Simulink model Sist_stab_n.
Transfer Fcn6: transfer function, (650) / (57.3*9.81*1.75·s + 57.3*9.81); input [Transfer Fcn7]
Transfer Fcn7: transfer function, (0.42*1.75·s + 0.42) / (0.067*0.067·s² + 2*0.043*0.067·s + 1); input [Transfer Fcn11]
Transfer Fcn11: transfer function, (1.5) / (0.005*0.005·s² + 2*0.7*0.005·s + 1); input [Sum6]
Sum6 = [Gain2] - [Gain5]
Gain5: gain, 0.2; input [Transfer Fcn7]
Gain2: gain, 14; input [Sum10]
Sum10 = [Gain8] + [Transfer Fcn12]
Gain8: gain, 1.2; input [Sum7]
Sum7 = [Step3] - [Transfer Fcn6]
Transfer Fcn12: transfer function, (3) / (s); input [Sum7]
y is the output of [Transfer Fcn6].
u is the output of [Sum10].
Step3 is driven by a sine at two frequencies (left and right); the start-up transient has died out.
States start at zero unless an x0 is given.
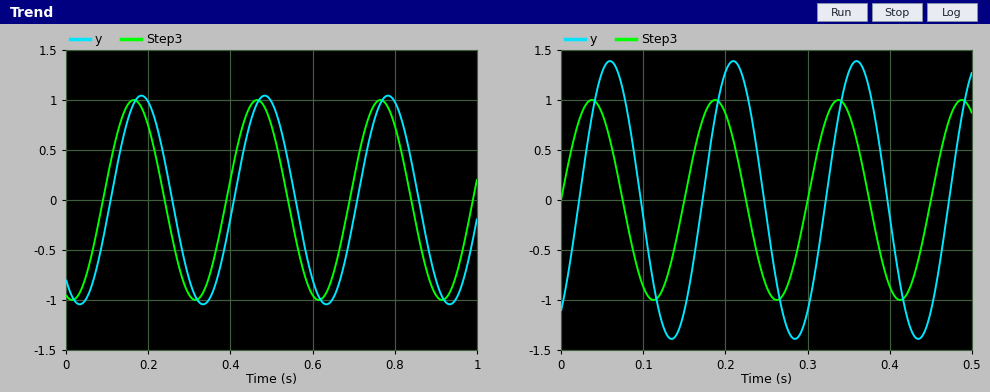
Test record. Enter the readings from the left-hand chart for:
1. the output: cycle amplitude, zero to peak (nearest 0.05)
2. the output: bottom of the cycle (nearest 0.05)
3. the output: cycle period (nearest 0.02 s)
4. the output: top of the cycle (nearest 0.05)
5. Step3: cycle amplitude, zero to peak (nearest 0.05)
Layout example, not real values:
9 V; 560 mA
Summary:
1.05; -1.05; 0.30 s; 1.05; 1.00
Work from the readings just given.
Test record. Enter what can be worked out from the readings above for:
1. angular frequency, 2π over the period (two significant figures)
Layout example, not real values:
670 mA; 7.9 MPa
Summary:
21 rad/s
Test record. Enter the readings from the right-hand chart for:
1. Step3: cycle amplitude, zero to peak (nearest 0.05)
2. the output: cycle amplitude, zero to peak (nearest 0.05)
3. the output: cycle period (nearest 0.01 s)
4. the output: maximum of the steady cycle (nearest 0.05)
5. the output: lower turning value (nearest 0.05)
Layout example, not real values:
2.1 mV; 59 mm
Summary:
1.00; 1.40; 0.15 s; 1.40; -1.40
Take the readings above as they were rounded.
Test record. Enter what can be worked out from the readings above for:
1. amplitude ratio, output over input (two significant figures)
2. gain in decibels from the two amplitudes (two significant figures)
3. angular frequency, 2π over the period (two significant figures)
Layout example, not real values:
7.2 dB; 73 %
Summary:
1.4; 2.9 dB; 42 rad/s
